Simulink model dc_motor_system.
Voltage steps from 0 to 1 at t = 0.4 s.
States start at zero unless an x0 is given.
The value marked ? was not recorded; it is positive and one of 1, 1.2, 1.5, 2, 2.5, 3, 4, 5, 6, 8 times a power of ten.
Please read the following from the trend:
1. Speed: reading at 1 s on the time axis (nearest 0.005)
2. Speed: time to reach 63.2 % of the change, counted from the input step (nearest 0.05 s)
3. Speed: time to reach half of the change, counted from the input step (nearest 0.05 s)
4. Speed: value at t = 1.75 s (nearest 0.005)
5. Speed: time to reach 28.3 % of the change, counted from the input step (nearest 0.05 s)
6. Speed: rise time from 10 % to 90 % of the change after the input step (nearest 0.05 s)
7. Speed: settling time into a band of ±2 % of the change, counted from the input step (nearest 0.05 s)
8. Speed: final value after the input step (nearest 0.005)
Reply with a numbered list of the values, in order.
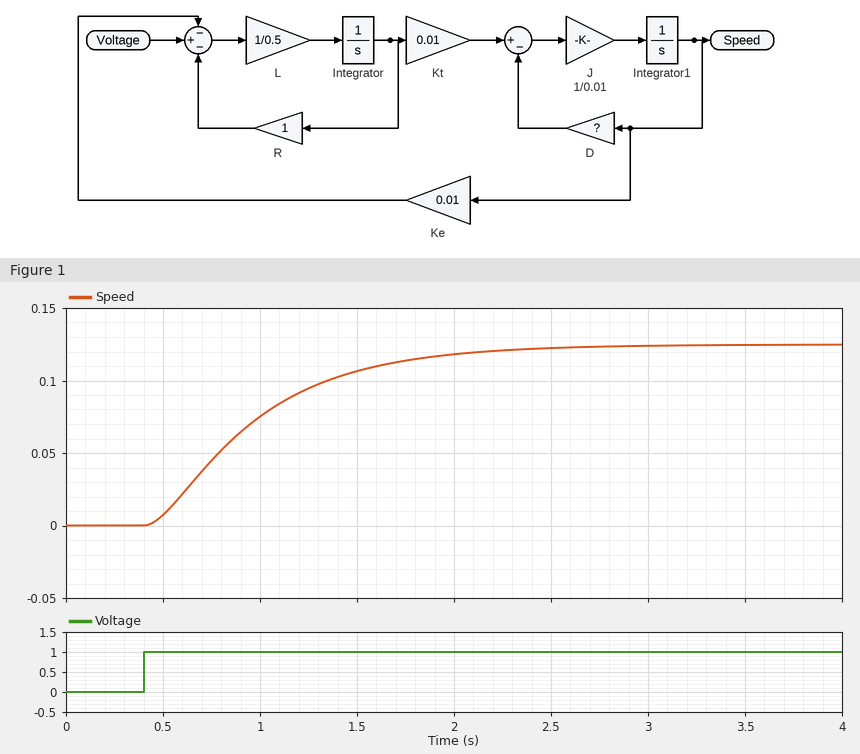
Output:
1. 0.075
2. 0.65 s
3. 0.50 s
4. 0.115
5. 0.30 s
6. 1.15 s
7. 2.10 s
8. 0.125
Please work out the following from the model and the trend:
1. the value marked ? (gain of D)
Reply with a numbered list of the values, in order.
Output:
1. 0.08
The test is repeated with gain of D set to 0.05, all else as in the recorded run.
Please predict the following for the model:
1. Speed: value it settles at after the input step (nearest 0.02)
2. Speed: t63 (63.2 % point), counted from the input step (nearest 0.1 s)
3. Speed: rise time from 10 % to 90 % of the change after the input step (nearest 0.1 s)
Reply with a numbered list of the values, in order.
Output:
1. 0.20
2. 0.7 s
3. 1.2 s
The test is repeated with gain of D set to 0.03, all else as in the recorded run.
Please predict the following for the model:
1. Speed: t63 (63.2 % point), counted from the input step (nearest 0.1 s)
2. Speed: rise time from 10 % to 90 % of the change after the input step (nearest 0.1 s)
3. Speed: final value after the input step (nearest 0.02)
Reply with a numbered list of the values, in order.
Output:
1. 0.9 s
2. 1.4 s
3. 0.34
